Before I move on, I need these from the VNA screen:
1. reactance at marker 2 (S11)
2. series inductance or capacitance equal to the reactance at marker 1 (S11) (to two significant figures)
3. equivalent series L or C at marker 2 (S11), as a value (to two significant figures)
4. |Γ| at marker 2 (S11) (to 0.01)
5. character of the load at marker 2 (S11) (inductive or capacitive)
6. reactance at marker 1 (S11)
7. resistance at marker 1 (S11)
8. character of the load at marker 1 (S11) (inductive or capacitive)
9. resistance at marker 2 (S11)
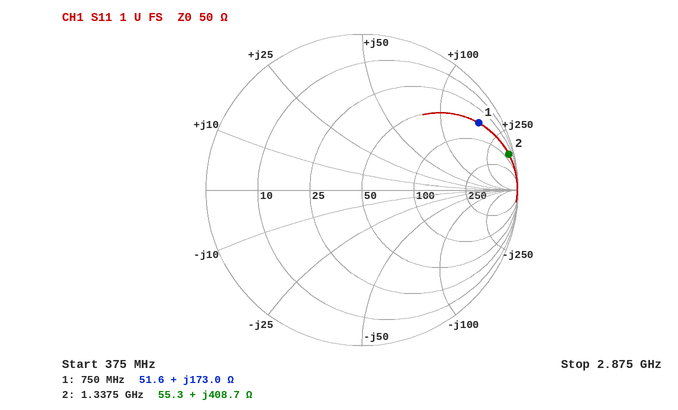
+408.7 Ω
37 nH
49 nH
0.97
inductive
+173.0 Ω
51.6 Ω
inductive
55.3 Ω
